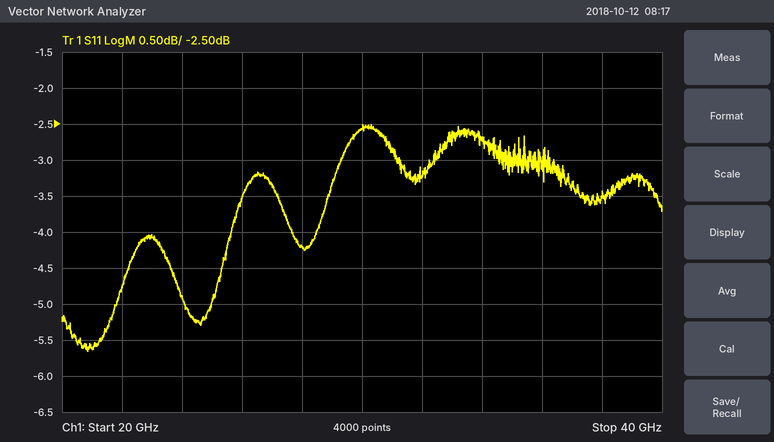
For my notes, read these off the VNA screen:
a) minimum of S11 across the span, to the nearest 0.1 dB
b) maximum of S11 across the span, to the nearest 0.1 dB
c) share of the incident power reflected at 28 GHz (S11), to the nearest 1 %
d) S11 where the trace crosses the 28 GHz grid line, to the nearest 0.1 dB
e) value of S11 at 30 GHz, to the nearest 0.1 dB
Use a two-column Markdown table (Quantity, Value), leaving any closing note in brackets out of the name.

| Quantity | Value |
|---|---|
| minimum of S11 across the span, to the nearest 0.1 dB | -5.7 dB |
| maximum of S11 across the span, to the nearest 0.1 dB | -2.5 dB |
| share of the incident power reflected at 28 GHz (S11), to the nearest 1 % | 38 % |
| S11 where the trace crosses the 28 GHz grid line, to the nearest 0.1 dB | -4.2 dB |
| value of S11 at 30 GHz, to the nearest 0.1 dB | -2.6 dB |
